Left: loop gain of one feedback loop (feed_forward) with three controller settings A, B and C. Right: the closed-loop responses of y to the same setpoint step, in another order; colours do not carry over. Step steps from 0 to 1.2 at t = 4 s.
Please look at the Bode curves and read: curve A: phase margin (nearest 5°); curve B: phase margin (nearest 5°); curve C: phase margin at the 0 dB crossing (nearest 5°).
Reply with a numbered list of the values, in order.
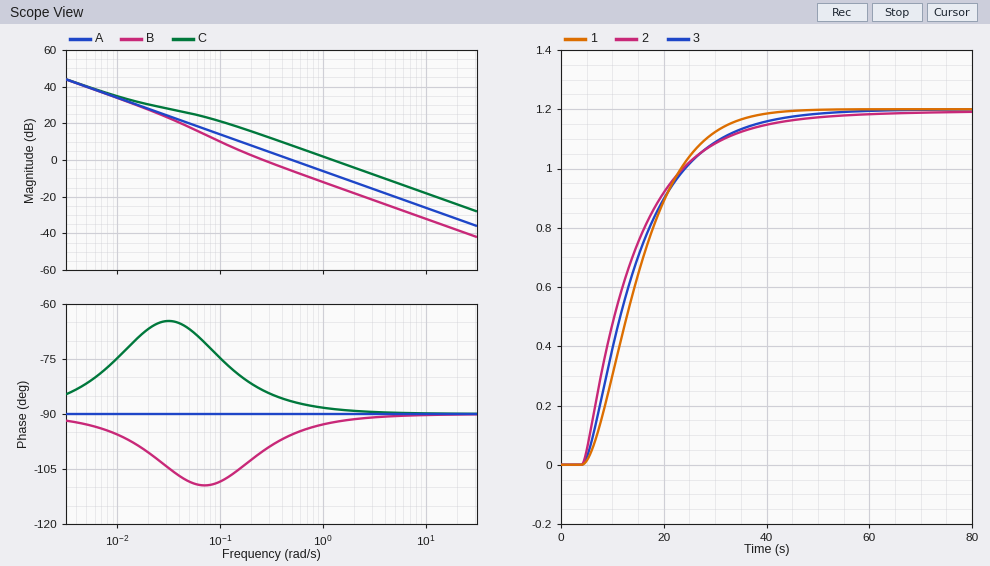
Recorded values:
1. 90°
2. 80°
3. 90°
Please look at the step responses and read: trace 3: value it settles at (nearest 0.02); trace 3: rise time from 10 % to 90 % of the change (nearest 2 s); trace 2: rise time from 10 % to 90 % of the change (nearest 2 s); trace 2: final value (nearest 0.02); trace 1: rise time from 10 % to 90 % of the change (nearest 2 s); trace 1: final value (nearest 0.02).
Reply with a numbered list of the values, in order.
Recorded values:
1. 1.20
2. 22 s
3. 24 s
4. 1.20
5. 20 s
6. 1.20
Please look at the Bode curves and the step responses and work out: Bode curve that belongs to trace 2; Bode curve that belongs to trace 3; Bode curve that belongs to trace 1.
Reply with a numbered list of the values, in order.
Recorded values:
1. C
2. A
3. B
